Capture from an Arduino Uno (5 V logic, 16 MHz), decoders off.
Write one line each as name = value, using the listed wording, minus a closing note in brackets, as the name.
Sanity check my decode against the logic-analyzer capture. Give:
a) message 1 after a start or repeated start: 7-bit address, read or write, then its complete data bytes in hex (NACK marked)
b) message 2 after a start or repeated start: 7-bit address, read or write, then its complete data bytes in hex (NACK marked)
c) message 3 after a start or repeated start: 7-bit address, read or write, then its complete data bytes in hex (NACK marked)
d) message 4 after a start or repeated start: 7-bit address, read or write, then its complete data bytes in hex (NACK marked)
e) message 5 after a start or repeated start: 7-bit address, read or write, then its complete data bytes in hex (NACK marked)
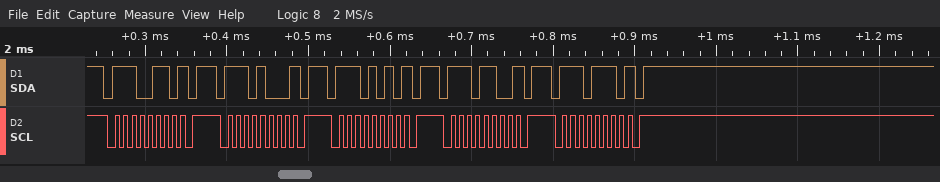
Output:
message 1 after a start or repeated start: 7-bit address, read or write, then its complete data bytes in hex = 0x73 write NACK
message 2 after a start or repeated start: 7-bit address, read or write, then its complete data bytes in hex = 0x74 write NACK
message 3 after a start or repeated start: 7-bit address, read or write, then its complete data bytes in hex = 0x75 write NACK
message 4 after a start or repeated start: 7-bit address, read or write, then its complete data bytes in hex = 0x76 write NACK
message 5 after a start or repeated start: 7-bit address, read or write, then its complete data bytes in hex = 0x77 write NACK
